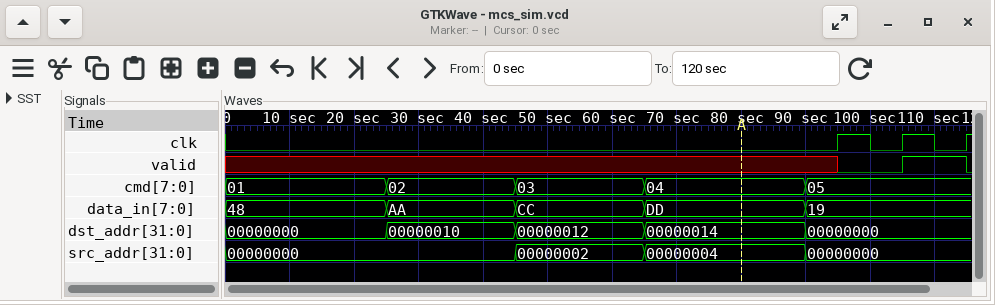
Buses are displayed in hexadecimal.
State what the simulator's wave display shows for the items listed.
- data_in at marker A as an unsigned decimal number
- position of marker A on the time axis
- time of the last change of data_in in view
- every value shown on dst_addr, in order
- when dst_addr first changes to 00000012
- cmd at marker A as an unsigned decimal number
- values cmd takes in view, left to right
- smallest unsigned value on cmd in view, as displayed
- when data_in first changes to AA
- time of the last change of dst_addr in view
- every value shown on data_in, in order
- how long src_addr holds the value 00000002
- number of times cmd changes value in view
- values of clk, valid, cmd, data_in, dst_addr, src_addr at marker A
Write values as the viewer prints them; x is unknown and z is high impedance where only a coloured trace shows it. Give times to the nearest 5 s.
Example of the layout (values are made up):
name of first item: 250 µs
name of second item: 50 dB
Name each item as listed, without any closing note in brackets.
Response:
data_in at marker A as an unsigned decimal number: 221
position of marker A on the time axis: 80 s
time of the last change of data_in in view: 90 s
every value shown on dst_addr, in order: 00000000, 00000010, 00000012, 00000014, 00000000
when dst_addr first changes to 00000012: 45 s
cmd at marker A as an unsigned decimal number: 4
values cmd takes in view, left to right: 01, 02, 03, 04, 05
smallest unsigned value on cmd in view, as displayed: 01
when data_in first changes to AA: 25 s
time of the last change of dst_addr in view: 90 s
every value shown on data_in, in order: 48, AA, CC, DD, 19
how long src_addr holds the value 00000002: 20 s
number of times cmd changes value in view: 4
values of clk, valid, cmd, data_in, dst_addr, src_addr at marker A: clk=0, valid=x, cmd=04, data_in=DD, dst_addr=00000014, src_addr=00000004
